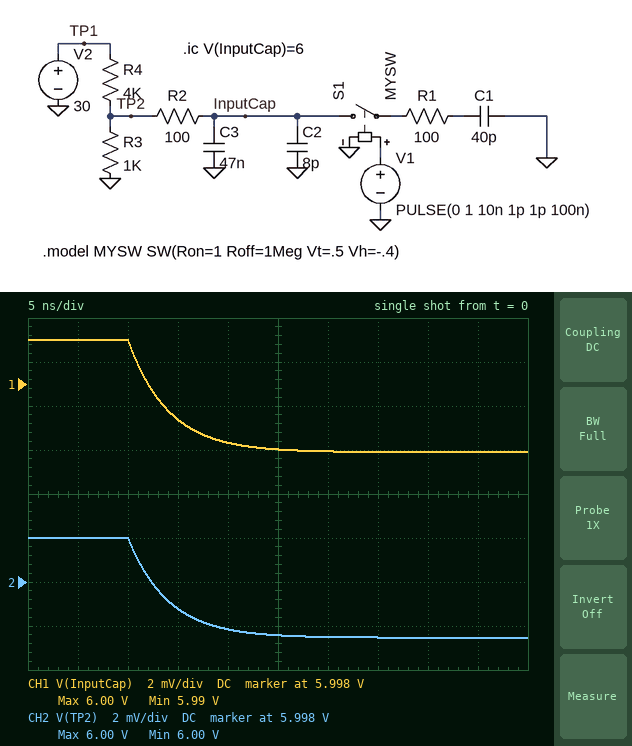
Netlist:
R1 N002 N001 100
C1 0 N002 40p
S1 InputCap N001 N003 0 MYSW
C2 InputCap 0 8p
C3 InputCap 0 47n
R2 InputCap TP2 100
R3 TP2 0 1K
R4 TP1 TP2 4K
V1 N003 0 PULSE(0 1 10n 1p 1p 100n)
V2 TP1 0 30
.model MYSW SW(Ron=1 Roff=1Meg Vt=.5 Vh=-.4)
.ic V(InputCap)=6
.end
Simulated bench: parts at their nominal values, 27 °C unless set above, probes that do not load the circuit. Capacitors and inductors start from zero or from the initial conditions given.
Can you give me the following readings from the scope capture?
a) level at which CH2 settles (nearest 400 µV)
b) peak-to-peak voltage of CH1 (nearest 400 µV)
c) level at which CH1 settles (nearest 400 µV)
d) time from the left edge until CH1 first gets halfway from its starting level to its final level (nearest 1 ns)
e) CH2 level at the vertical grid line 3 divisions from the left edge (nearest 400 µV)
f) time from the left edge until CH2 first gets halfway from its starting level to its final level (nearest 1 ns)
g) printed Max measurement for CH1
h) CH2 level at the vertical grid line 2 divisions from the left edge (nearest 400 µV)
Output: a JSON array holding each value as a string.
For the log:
["5.9956 V", "5.2 mV", "5.9948 V", "13 ns", "5.9968 V", "13 ns", "6.00 V", "6.0000 V"]
